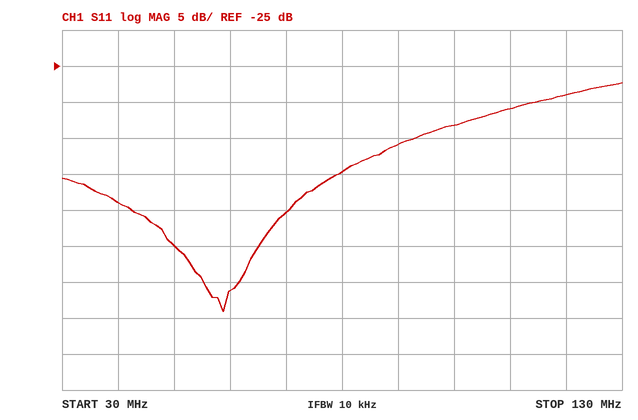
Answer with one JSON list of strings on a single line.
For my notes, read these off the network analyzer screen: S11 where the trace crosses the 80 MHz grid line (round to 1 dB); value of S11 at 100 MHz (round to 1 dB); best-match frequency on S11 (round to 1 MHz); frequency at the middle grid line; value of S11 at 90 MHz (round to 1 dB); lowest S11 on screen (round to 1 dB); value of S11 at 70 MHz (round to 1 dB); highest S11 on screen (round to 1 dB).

["-40 dB", "-33 dB", "59 MHz", "80 MHz", "-36 dB", "-59 dB", "-45 dB", "-27 dB"]
